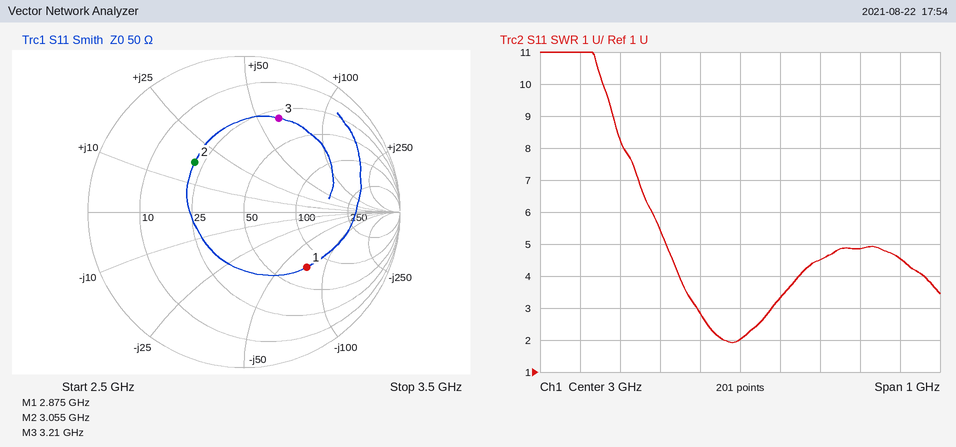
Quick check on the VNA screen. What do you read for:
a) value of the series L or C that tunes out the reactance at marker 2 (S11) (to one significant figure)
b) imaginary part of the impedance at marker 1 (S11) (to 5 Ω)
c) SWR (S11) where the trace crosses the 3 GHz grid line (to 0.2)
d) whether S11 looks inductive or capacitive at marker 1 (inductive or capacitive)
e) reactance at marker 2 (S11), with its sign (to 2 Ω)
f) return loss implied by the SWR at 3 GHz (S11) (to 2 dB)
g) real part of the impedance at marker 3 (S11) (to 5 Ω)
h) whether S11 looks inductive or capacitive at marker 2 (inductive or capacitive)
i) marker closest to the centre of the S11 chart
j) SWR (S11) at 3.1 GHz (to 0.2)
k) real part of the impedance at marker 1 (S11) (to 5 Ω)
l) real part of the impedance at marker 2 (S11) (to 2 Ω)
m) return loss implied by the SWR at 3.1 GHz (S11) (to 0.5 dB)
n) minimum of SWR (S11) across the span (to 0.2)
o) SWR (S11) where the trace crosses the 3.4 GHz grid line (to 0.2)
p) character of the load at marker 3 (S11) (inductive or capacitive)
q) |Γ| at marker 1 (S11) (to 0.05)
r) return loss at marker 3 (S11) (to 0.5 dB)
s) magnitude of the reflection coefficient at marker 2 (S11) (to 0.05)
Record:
3 pF
-75 Ω
2.0
capacitive
+18 Ω
10 dB
30 Ω
inductive
marker 2
3.4
75 Ω
22 Ω
5.5 dB
2.0
4.6
inductive
0.55
4.0 dB
0.45
